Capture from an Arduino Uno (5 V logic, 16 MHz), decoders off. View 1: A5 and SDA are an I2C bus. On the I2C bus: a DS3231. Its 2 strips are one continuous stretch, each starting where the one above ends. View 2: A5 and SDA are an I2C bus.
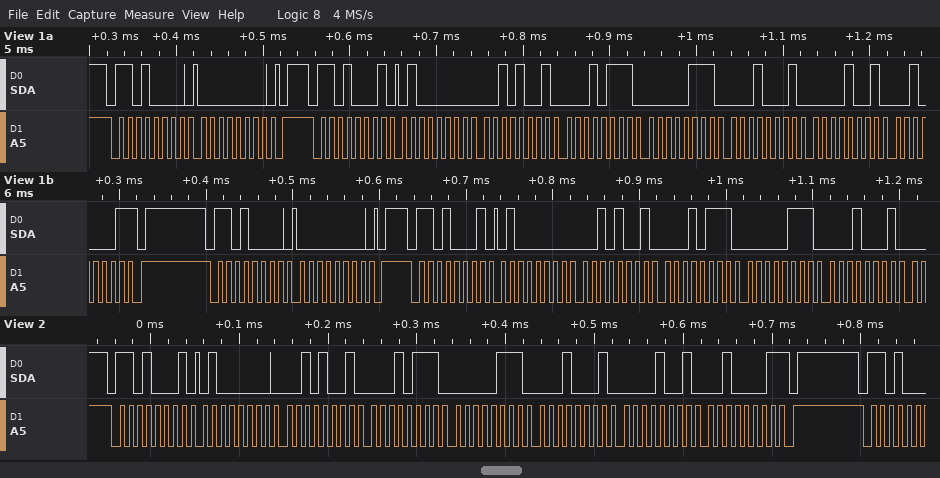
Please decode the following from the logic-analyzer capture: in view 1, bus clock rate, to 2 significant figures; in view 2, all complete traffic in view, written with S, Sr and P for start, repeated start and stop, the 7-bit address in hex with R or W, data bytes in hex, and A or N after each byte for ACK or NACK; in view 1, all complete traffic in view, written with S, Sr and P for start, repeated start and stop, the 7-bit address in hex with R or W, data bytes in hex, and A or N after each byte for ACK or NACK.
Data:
100 kHz
S 68R A 40 A 29 A 17 A 07 A 11 A 09 A 21 N P
S 68W A 00 A P S 68R A 40 A 29 A 17 A 07 A 11 A 09 A 21 N P S 68W A 00 A P S 68R A 40 A 29 A 17 A 07 A 11 A
